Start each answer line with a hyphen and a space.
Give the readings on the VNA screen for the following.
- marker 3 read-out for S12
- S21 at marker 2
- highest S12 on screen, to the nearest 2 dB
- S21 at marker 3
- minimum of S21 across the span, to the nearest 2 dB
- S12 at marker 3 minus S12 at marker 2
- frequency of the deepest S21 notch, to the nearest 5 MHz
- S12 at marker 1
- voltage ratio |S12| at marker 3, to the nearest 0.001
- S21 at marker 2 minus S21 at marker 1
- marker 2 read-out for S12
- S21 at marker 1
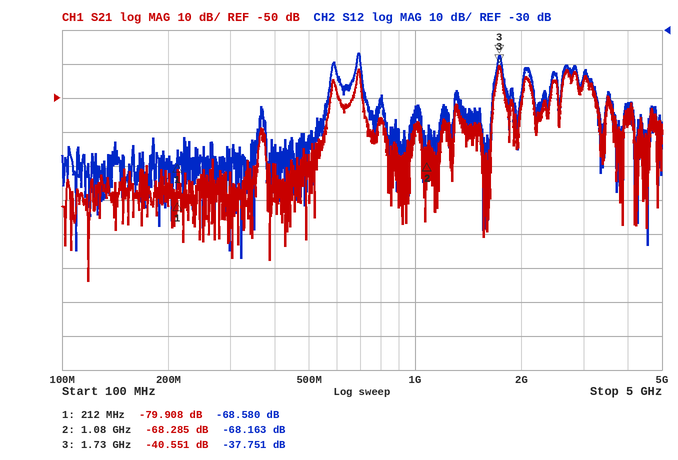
- -37.751 dB
- -68.285 dB
- -36 dB
- -40.551 dB
- -104 dB
- 30.412 dB
- 120 MHz
- -68.580 dB
- 0.013
- 11.623 dB
- -68.163 dB
- -79.908 dB
